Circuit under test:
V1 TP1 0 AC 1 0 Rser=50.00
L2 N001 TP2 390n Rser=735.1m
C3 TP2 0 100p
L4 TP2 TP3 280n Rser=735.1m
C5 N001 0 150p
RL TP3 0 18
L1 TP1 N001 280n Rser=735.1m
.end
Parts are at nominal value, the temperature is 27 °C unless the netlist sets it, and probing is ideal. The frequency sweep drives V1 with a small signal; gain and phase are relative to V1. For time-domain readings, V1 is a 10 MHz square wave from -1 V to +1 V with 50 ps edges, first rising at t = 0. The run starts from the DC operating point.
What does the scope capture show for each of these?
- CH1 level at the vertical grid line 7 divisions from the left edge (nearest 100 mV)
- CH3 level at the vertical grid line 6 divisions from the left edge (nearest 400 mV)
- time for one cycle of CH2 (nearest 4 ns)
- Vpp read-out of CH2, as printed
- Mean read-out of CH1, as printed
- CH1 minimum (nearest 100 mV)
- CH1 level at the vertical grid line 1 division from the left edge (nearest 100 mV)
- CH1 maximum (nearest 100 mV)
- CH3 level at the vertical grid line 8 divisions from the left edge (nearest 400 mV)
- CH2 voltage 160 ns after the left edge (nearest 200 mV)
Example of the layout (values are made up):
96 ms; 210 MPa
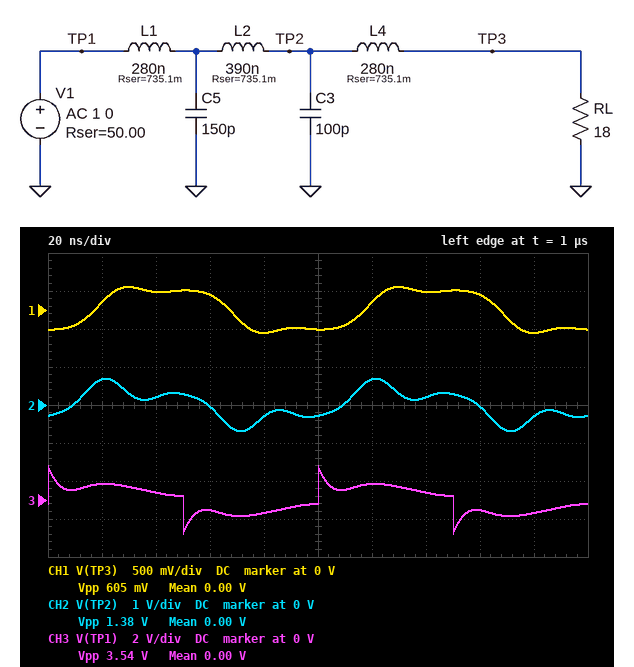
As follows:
200 mV; 800 mV; 100 ns; 1.38 V; 0.00 V; -300 mV; 100 mV; 300 mV; -400 mV; 0 V
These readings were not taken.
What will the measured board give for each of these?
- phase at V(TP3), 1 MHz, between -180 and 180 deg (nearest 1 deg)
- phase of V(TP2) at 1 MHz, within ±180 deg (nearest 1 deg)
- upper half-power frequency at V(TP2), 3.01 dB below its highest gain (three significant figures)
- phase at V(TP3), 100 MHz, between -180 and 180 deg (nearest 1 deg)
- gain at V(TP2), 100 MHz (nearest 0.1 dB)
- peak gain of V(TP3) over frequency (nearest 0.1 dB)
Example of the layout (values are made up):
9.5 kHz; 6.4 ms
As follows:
-6 deg; -1 deg; 44.6 MHz; -66 deg; -46.1 dB; -11.8 dB
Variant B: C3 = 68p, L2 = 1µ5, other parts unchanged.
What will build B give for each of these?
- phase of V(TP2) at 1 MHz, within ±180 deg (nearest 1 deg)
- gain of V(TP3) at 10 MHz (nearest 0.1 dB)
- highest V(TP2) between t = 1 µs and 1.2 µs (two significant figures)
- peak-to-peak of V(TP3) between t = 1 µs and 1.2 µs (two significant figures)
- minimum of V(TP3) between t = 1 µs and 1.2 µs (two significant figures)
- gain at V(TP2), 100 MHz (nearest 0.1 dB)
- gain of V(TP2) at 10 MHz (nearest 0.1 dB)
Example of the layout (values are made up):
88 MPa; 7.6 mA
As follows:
-6 deg; -16.0 dB; 310 mV; 400 mV; -200 mV; -54.8 dB; -12.9 dB
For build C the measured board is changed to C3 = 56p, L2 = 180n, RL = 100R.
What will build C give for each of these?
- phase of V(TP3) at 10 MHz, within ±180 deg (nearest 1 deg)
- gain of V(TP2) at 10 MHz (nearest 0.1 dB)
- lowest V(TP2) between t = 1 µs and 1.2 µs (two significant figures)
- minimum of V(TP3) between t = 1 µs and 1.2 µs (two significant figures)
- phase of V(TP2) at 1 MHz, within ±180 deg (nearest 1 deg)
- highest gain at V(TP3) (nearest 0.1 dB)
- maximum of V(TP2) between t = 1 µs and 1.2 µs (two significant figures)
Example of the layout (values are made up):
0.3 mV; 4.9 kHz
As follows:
-44 deg; -3.4 dB; -790 mV; -760 mV; -3 deg; -3.6 dB; 790 mV
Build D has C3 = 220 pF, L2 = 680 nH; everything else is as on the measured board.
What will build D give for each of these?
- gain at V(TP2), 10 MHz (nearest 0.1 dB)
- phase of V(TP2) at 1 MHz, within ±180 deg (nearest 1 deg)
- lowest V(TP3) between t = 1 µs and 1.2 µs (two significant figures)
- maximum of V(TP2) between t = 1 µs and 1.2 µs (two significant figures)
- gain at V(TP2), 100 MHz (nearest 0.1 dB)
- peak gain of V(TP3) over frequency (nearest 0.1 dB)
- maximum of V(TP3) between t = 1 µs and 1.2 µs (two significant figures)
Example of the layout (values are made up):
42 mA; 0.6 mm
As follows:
-9.2 dB; -3 deg; -340 mV; 620 mV; -58.9 dB; -10.8 dB; 340 mV
